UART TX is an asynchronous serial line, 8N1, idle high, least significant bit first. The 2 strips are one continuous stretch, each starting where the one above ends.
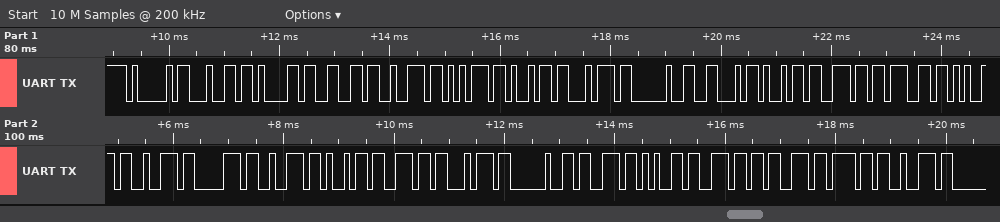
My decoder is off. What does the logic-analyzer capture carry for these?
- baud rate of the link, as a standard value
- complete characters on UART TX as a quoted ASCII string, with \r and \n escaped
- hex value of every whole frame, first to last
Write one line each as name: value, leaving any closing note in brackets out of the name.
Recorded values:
baud rate of the link, as a standard value: 9600 baud
complete characters on UART TX as a quoted ASCII string, with \r and \n escaped: "Adafruit Fingerprint sensor"
hex value of every whole frame, first to last: 41 64 61 66 72 75 69 74 20 46 69 6E 67 65 72 70 72 69 6E 74 20 73 65 6E 73 6F 72
